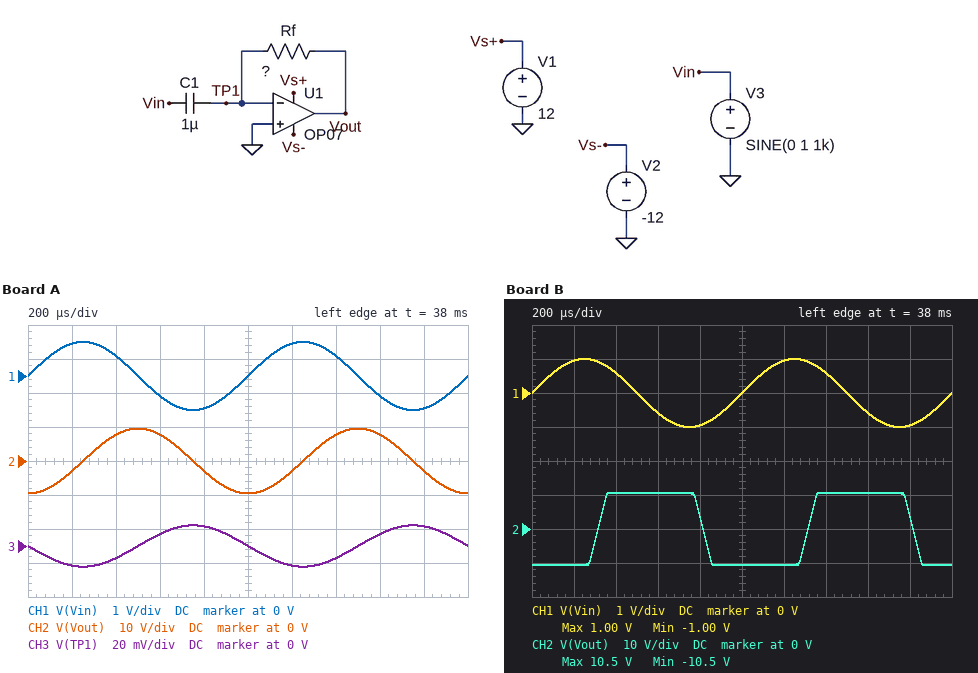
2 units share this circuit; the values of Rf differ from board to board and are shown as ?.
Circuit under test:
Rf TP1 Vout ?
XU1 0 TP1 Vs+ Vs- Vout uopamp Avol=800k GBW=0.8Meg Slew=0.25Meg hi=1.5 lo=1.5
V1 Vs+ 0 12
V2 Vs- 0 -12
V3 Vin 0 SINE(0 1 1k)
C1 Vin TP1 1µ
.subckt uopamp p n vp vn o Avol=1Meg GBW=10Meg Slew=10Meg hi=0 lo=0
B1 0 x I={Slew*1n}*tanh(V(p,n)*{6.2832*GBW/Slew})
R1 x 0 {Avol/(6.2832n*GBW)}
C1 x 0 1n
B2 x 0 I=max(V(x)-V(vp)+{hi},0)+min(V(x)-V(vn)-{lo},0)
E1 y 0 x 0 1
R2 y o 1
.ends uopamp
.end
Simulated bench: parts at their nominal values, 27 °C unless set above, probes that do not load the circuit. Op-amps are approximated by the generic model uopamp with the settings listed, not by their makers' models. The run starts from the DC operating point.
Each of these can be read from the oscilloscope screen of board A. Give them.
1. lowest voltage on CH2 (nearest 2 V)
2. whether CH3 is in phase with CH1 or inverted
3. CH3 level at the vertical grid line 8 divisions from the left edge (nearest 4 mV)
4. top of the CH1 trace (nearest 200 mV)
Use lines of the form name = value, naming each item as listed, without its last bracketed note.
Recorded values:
lowest voltage on CH2 = -10 V
whether CH3 is in phase with CH1 or inverted = inverted
CH3 level at the vertical grid line 8 divisions from the left edge = 8 mV
top of the CH1 trace = 1.0 V
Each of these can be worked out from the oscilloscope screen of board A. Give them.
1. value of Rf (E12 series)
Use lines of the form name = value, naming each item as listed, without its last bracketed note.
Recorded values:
value of Rf = 1.5 kΩ
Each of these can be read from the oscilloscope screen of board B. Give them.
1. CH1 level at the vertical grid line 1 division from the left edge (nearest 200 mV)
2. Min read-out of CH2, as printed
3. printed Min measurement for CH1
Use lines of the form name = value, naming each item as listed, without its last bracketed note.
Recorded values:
CH1 level at the vertical grid line 1 division from the left edge = 1.0 V
Min read-out of CH2, as printed = -10.5 V
printed Min measurement for CH1 = -1.00 V
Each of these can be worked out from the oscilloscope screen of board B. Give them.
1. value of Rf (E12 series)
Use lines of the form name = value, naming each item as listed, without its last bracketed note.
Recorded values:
value of Rf = 2.2 kΩ
